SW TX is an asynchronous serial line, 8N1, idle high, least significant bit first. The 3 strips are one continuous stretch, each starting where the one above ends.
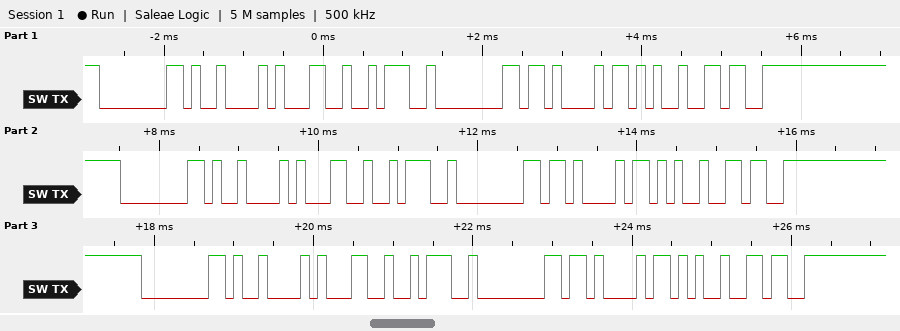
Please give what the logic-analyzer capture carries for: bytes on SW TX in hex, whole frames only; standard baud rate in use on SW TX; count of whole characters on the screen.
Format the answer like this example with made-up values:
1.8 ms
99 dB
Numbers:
80 09 31 3A 80 0B 2B 36 80 09 31 3A 80 0B 2B 36 80 09 31 3A 80 0B 2B 36
9600 baud
24
